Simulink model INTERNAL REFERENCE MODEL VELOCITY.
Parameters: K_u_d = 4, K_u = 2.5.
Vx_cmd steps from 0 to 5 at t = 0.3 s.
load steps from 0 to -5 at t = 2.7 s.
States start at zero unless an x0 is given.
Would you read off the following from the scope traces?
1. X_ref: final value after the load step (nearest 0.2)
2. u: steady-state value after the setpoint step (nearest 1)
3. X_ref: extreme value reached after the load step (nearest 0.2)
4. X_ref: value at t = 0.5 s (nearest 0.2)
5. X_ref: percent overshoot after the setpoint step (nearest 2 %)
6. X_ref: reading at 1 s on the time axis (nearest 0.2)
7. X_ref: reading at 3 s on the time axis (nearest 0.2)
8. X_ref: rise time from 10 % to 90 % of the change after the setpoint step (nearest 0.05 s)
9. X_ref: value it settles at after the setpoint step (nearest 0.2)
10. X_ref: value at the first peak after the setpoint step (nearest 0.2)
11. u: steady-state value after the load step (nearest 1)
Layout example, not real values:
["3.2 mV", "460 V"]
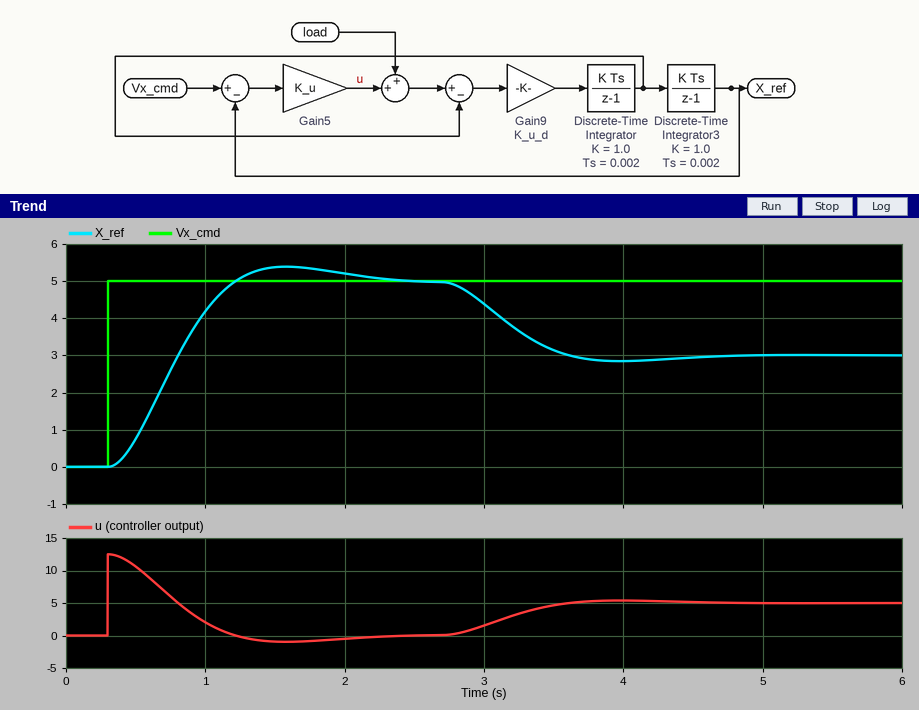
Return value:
["3.0", "0", "2.8", "0.8", "8 %", "4.2", "4.4", "0.60 s", "5.0", "5.4", "5"]
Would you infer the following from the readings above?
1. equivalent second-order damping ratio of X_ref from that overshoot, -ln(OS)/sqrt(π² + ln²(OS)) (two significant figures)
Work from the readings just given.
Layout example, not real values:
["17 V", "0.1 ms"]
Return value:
["0.63"]
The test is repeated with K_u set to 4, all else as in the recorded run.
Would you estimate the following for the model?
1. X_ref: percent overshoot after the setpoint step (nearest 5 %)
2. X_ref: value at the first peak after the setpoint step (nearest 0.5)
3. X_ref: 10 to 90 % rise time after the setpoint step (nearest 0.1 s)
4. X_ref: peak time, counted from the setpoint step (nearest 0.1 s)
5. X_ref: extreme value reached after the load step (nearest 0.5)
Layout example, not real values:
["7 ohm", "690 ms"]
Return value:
["15 %", "6.0", "0.4 s", "0.9 s", "3.5"]
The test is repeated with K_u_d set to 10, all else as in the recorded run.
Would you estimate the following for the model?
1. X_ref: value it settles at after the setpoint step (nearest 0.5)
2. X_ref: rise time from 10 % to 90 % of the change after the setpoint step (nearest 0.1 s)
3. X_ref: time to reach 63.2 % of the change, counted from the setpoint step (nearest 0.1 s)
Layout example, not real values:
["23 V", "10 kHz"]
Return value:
["5.0", "0.7 s", "0.4 s"]
